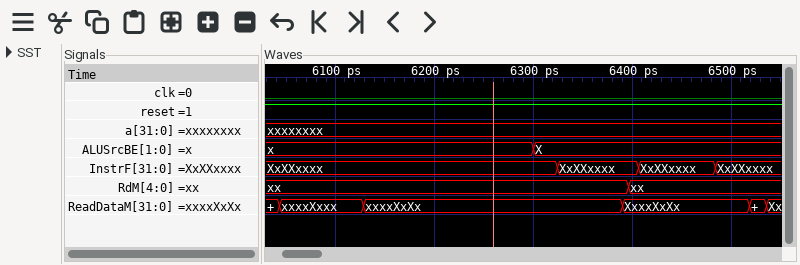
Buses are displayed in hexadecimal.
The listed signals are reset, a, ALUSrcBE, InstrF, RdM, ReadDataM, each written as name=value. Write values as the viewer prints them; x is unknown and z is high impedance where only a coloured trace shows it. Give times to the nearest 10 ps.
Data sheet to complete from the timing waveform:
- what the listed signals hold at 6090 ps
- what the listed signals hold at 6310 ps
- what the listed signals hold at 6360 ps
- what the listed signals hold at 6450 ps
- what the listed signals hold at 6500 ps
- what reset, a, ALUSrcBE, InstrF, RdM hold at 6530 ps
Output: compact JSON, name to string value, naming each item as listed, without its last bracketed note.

{"what the listed signals hold at 6090 ps": "reset=1, a=xxxxxxxx, ALUSrcBE=x, InstrF=XxXXxxxx, RdM=xx, ReadDataM=xxxxXxxx", "what the listed signals hold at 6310 ps": "reset=1, a=xxxxxxxx, ALUSrcBE=X, InstrF=XxXXxxxx, RdM=xx, ReadDataM=xxxxXxXx", "what the listed signals hold at 6360 ps": "reset=1, a=xxxxxxxx, ALUSrcBE=X, InstrF=XxXXxxxx, RdM=xx, ReadDataM=xxxxXxXx", "what the listed signals hold at 6450 ps": "reset=1, a=xxxxxxxx, ALUSrcBE=X, InstrF=XxXXxxxx, RdM=xx, ReadDataM=XxxxXxXx", "what the listed signals hold at 6500 ps": "reset=1, a=xxxxxxxx, ALUSrcBE=X, InstrF=XxXXxxxx, RdM=xx, ReadDataM=XxxxXxXx", "what reset, a, ALUSrcBE, InstrF, RdM hold at 6530 ps": "reset=1, a=xxxxxxxx, ALUSrcBE=X, InstrF=XxXXxxxx, RdM=xx"}
